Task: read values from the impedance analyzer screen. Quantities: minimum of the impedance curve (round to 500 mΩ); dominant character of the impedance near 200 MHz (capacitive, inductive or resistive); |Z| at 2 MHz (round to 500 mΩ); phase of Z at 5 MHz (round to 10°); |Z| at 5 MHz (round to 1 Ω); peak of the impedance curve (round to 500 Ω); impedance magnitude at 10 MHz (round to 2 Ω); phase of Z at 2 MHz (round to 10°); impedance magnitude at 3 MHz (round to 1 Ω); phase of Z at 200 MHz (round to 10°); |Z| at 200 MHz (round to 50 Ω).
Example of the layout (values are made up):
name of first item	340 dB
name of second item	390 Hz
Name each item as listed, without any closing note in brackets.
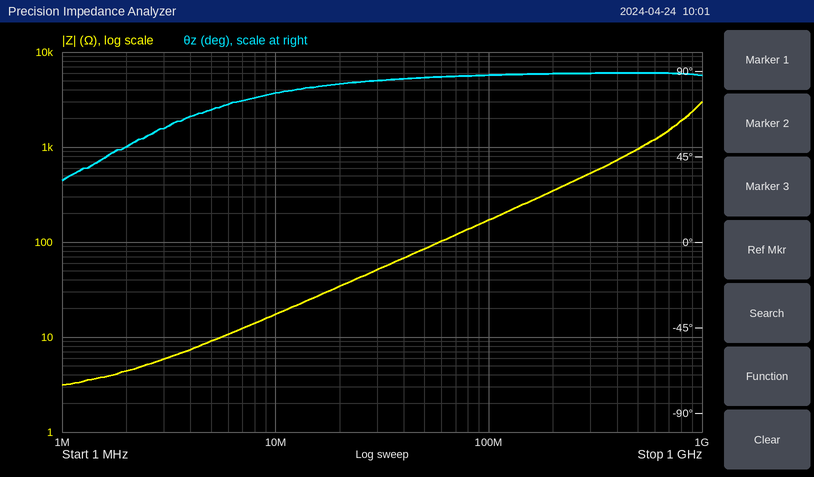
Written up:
minimum of the impedance curve	3.0 Ω
dominant character of the impedance near 200 MHz	inductive
|Z| at 2 MHz	4.5 Ω
phase of Z at 5 MHz	70°
|Z| at 5 MHz	9 Ω
peak of the impedance curve	3.0 kΩ
impedance magnitude at 10 MHz	18 Ω
phase of Z at 2 MHz	50°
impedance magnitude at 3 MHz	6 Ω
phase of Z at 200 MHz	90°
|Z| at 200 MHz	350 Ω
